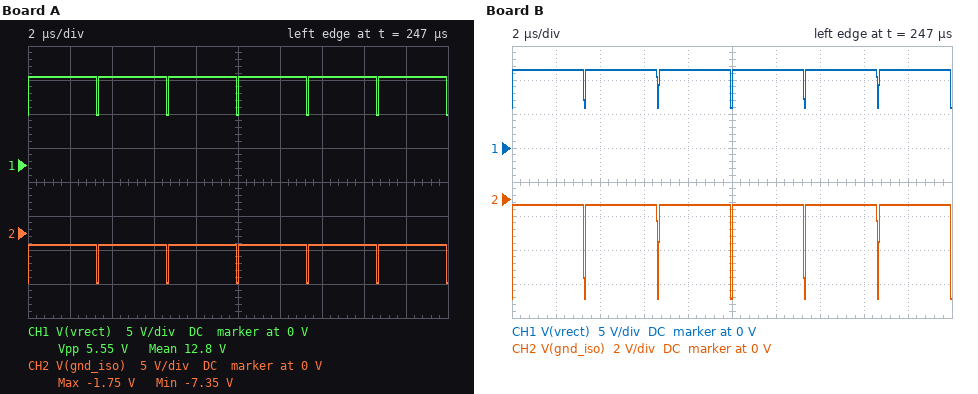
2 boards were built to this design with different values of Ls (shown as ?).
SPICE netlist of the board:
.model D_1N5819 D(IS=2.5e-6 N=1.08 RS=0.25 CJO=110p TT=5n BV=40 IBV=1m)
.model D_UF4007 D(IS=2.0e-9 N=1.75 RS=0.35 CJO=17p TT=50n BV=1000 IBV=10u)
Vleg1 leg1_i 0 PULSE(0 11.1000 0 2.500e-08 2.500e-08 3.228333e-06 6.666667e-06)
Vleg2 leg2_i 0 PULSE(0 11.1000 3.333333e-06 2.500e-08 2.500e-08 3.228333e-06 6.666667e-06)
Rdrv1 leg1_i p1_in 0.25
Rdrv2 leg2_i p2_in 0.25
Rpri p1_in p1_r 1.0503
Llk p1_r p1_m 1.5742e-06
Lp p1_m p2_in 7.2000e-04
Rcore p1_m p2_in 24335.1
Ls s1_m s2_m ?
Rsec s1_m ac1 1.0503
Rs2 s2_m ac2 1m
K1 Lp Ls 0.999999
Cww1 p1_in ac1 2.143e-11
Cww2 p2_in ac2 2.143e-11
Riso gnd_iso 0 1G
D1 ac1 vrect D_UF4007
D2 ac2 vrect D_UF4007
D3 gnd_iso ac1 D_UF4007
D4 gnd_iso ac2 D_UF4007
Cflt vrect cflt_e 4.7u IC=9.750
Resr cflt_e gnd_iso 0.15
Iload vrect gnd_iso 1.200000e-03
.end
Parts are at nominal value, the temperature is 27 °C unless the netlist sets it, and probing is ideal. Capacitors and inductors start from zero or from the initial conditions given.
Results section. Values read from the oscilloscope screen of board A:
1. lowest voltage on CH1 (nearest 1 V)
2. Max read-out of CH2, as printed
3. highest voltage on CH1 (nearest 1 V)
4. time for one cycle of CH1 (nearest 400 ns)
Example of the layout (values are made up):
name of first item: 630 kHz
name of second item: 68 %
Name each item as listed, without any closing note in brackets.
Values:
lowest voltage on CH1: 7 V
Max read-out of CH2, as printed: -1.75 V
highest voltage on CH1: 13 V
time for one cycle of CH1: 3.2 µs
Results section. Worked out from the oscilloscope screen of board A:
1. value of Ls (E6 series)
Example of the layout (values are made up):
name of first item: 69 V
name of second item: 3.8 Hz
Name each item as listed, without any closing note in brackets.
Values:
value of Ls: 1.5 mH
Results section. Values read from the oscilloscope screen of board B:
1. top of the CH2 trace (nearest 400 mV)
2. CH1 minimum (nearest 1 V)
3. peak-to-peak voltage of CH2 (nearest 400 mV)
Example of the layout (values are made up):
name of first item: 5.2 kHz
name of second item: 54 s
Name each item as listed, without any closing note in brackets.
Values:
top of the CH2 trace: -400 mV
CH1 minimum: 6 V
peak-to-peak voltage of CH2: 5.6 V
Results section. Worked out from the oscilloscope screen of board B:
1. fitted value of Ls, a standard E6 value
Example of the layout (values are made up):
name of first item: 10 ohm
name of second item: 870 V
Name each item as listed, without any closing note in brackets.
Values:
fitted value of Ls, a standard E6 value: 1 mH
